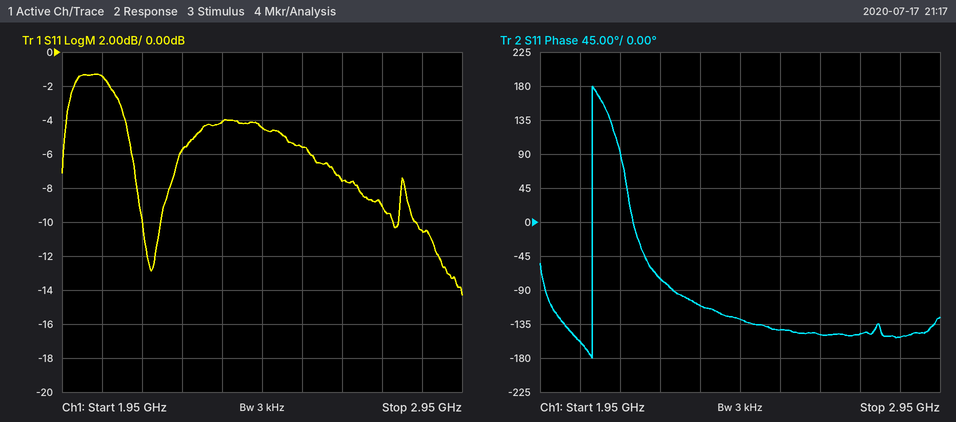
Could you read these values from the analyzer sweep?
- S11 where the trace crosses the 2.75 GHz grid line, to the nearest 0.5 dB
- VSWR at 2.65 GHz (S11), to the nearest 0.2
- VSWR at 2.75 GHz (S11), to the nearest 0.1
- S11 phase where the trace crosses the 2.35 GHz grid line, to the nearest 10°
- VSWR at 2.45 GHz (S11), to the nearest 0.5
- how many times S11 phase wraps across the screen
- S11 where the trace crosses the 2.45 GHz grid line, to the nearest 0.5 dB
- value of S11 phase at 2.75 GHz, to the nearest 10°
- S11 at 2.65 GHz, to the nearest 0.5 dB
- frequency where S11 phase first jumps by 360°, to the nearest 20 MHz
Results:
-9.0 dB
2.4
2.1
-110°
4.0
1
-4.5 dB
-150°
-7.5 dB
2.08 GHz
